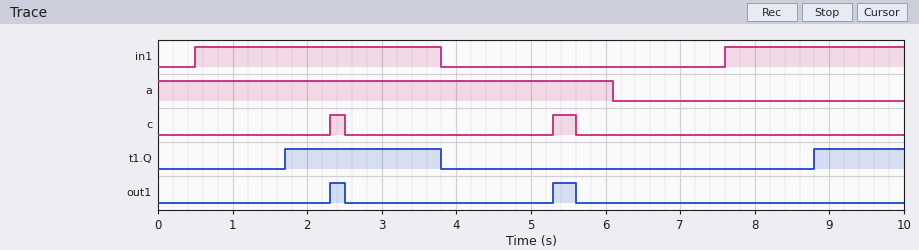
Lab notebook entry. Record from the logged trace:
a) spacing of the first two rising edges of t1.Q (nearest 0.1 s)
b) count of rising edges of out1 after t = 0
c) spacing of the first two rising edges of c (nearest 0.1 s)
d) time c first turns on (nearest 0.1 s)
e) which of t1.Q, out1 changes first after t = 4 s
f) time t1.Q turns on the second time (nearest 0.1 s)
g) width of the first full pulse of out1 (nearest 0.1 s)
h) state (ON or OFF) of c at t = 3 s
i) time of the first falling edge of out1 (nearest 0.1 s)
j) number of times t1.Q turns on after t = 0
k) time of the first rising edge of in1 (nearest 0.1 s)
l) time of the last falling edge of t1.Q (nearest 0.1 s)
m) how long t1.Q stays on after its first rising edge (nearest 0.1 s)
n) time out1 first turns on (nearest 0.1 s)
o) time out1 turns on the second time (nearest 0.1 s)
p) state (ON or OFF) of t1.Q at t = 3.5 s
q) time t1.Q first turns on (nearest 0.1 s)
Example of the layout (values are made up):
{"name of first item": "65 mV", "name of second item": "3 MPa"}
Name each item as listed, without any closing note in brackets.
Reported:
{"spacing of the first two rising edges of t1.Q": "7.1 s", "count of rising edges of out1 after t = 0": "2", "spacing of the first two rising edges of c": "3.0 s", "time c first turns on": "2.3 s", "which of t1.Q, out1 changes first after t = 4 s": "out1", "time t1.Q turns on the second time": "8.8 s", "width of the first full pulse of out1": "0.2 s", "state (ON or OFF) of c at t = 3 s": "OFF", "time of the first falling edge of out1": "2.5 s", "number of times t1.Q turns on after t = 0": "2", "time of the first rising edge of in1": "0.5 s", "time of the last falling edge of t1.Q": "3.8 s", "how long t1.Q stays on after its first rising edge": "2.1 s", "time out1 first turns on": "2.3 s", "time out1 turns on the second time": "5.3 s", "state (ON or OFF) of t1.Q at t = 3.5 s": "ON", "time t1.Q first turns on": "1.7 s"}
